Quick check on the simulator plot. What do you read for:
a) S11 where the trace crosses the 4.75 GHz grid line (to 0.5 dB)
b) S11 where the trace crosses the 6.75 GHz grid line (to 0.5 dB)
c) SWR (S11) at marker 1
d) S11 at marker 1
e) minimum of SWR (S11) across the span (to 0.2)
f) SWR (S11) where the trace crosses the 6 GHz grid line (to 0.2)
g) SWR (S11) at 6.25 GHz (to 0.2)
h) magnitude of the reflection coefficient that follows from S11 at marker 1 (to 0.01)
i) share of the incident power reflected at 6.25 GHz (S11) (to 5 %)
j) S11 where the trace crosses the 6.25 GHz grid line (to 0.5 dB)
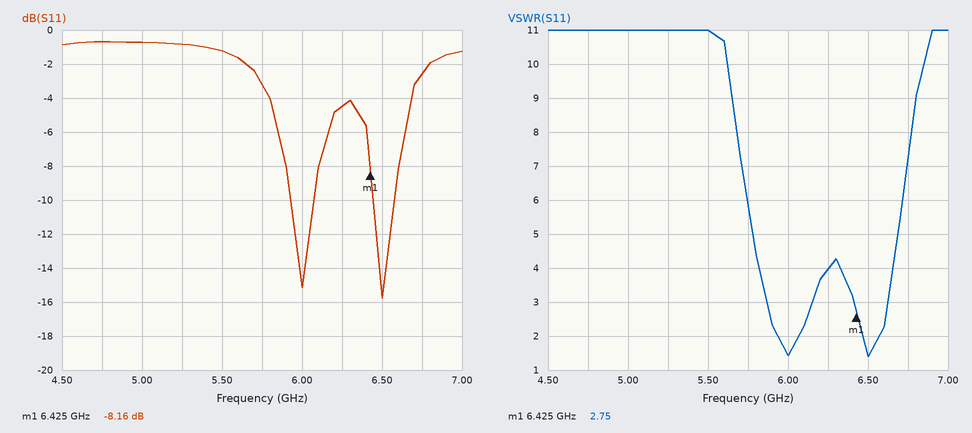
-0.5 dB
-2.5 dB
2.75
-8.16 dB
1.4
1.4
4.0
0.39
35 %
-4.5 dB
